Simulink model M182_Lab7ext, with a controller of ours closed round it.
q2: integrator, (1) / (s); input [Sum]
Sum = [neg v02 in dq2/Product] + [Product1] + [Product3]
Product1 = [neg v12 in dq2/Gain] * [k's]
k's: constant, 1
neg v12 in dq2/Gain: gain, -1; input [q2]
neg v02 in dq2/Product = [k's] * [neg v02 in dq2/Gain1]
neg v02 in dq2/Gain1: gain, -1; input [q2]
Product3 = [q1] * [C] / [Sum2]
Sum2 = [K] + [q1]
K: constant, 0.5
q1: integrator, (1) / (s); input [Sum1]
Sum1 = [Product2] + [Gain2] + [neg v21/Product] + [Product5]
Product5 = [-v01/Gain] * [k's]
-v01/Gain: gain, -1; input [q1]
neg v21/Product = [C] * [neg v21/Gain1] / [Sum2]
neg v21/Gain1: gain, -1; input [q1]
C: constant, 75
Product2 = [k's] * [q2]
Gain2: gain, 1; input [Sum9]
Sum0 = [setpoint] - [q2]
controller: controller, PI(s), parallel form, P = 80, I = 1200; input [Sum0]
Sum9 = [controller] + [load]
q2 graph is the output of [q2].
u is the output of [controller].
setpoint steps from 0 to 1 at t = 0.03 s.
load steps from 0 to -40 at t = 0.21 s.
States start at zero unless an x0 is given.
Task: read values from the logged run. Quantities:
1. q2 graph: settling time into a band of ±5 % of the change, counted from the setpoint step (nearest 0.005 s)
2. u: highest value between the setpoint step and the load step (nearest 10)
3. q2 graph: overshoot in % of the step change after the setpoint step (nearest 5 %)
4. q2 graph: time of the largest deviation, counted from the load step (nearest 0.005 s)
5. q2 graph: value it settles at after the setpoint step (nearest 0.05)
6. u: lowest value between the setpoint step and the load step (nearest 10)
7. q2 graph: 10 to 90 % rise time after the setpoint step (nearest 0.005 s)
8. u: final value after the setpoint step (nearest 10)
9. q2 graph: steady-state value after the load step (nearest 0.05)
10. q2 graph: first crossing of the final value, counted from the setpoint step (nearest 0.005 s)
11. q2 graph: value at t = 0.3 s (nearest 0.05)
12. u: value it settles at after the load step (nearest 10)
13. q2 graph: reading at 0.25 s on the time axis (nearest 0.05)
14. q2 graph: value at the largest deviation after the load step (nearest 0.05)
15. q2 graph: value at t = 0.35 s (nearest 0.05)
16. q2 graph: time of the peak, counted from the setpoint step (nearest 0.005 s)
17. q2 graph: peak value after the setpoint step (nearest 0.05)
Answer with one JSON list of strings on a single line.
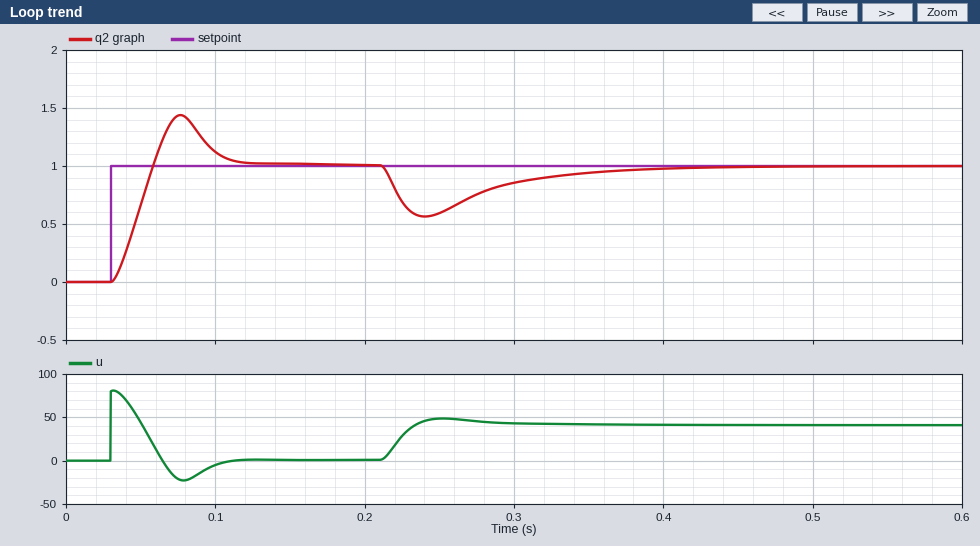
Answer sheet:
["0.080 s", "80", "45 %", "0.030 s", "1.00", "-20", "0.020 s", "0", "1.00", "0.030 s", "0.85", "40", "0.60", "0.55", "0.95", "0.045 s", "1.45"]
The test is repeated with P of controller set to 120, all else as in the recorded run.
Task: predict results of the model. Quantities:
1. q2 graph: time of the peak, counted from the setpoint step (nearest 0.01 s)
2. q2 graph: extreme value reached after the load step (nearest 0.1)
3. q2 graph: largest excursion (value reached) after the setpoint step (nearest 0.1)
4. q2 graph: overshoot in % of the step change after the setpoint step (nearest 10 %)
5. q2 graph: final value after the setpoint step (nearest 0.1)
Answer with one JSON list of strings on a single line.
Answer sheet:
["0.04 s", "0.7", "1.5", "50 %", "1.0"]
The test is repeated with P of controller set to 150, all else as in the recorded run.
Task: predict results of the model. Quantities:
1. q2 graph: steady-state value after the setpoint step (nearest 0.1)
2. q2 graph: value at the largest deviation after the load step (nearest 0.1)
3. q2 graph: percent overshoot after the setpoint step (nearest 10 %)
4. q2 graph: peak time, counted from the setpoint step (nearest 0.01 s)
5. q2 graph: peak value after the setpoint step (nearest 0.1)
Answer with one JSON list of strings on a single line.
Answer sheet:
["1.0", "0.7", "50 %", "0.04 s", "1.5"]
